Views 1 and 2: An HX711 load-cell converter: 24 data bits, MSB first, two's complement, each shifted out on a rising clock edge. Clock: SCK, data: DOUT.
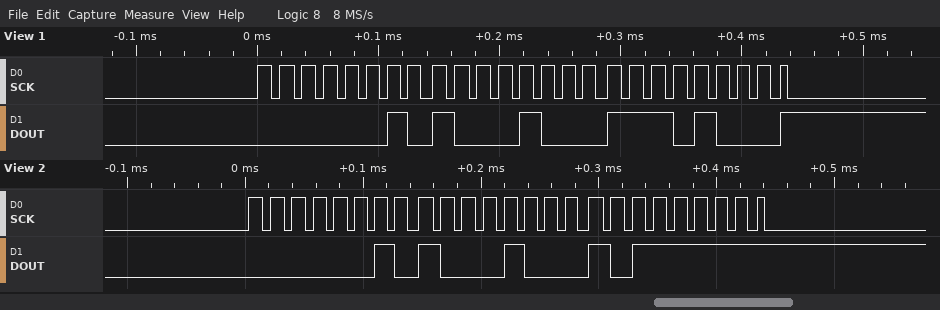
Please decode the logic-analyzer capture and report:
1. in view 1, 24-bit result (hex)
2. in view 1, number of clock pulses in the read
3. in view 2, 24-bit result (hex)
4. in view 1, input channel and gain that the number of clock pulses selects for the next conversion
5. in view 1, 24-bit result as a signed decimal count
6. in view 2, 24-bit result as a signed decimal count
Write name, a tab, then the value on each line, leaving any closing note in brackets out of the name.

in view 1, 24-bit result	0x0288E8
in view 1, number of clock pulses in the read	25
in view 2, 24-bit result	0x0288BF
in view 1, input channel and gain that the number of clock pulses selects for the next conversion	channel A, gain 128
in view 1, 24-bit result as a signed decimal count	166120
in view 2, 24-bit result as a signed decimal count	166079
